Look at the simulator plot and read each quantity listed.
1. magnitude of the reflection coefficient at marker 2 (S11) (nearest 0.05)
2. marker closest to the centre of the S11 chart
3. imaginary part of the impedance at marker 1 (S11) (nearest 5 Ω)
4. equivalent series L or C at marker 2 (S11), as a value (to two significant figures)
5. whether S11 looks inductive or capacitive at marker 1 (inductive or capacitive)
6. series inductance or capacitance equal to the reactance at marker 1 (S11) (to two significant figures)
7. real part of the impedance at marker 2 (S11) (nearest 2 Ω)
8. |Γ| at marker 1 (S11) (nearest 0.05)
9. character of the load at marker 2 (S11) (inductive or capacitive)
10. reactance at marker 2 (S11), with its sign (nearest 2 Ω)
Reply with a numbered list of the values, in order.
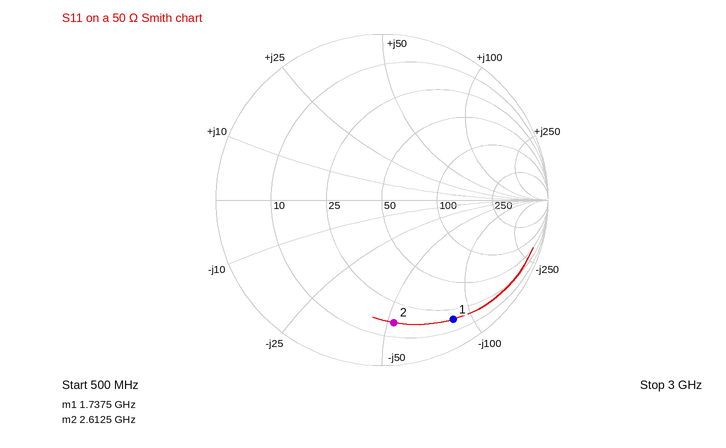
1. 0.75
2. marker 2
3. -85 Ω
4. 1.2 pF
5. capacitive
6. 1.1 pF
7. 16 Ω
8. 0.85
9. capacitive
10. -52 Ω
